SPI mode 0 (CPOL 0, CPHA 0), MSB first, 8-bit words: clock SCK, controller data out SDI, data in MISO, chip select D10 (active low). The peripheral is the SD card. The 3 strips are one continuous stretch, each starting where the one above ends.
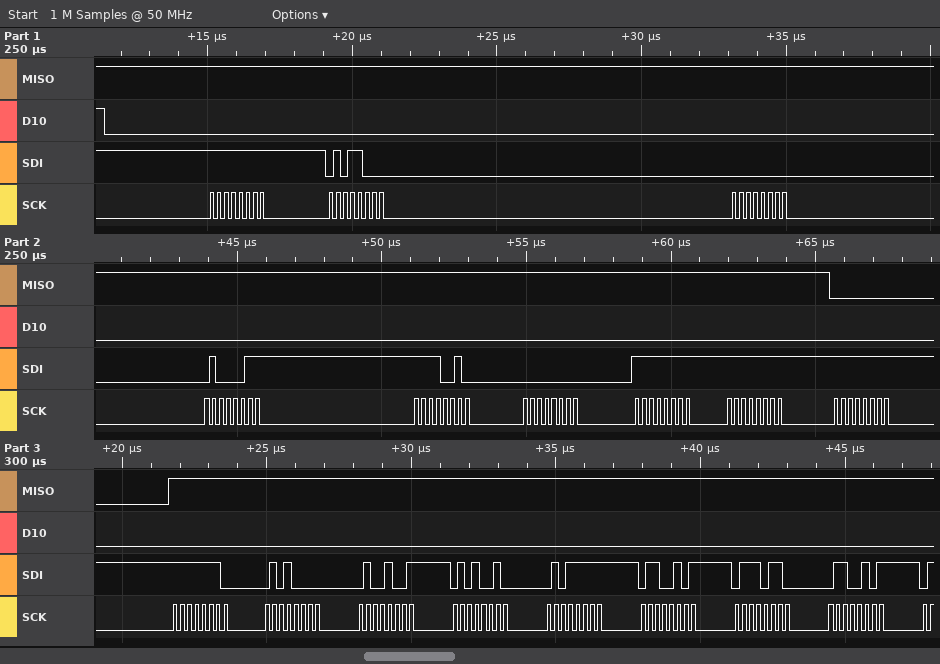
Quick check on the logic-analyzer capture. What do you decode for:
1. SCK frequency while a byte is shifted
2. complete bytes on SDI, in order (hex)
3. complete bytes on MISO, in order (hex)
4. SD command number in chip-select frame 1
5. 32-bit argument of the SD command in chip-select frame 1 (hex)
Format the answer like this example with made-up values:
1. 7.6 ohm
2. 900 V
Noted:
1. 4 MHz
2. FF 58 00 43 F2 00 FF FF FF FE 50 49 52 5F 65 76 65
3. FF FF FF FF FF FF FF FF 00 FF FF FF FF FF FF FF FF
4. CMD24
5. 0x0043F200
